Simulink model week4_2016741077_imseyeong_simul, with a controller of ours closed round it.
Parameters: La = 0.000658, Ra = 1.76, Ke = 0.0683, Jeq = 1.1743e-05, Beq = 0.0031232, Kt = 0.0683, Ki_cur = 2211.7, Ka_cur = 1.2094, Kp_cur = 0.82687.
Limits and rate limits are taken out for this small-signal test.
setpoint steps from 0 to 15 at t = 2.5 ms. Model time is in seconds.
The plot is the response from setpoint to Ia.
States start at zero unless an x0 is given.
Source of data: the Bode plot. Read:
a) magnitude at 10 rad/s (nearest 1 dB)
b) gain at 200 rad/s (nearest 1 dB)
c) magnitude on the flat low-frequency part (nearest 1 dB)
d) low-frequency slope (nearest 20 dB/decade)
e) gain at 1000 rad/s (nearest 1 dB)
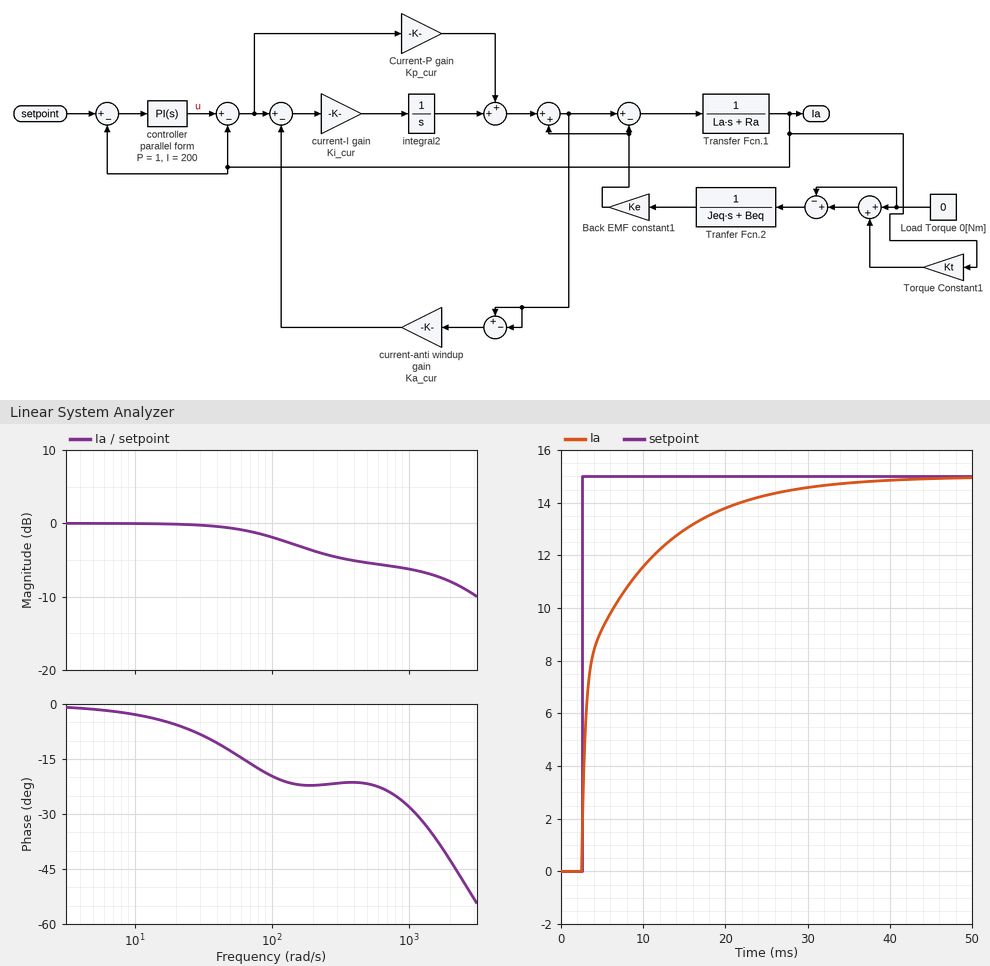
0 dB
-4 dB
0 dB
0 dB/decade
-6 dB
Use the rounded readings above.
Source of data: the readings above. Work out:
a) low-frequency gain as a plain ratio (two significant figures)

1.0
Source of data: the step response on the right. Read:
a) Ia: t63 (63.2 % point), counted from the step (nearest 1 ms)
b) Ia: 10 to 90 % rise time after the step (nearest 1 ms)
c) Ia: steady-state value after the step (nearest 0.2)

3 ms
15 ms
15.0
